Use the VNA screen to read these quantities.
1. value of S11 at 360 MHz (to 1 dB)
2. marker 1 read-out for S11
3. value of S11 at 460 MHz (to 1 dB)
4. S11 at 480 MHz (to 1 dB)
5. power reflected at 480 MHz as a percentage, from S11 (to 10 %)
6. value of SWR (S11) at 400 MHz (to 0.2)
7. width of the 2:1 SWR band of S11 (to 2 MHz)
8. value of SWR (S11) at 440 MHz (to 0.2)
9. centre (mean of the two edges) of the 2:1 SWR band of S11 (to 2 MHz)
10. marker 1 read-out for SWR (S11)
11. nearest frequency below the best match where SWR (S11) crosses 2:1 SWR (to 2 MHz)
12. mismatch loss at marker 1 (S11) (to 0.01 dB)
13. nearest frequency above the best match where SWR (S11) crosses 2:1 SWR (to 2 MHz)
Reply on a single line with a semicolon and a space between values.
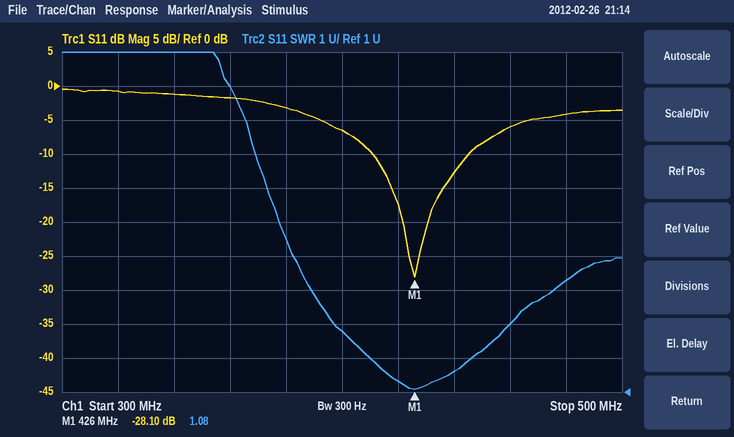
-2 dB; -28.10 dB; -6 dB; -4 dB; 40 %; 2.8; 36 MHz; 1.6; 428 MHz; 1.08; 410 MHz; 0.01 dB; 446 MHz
